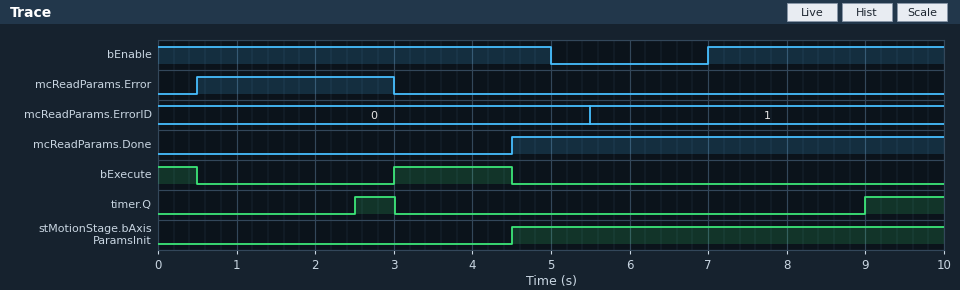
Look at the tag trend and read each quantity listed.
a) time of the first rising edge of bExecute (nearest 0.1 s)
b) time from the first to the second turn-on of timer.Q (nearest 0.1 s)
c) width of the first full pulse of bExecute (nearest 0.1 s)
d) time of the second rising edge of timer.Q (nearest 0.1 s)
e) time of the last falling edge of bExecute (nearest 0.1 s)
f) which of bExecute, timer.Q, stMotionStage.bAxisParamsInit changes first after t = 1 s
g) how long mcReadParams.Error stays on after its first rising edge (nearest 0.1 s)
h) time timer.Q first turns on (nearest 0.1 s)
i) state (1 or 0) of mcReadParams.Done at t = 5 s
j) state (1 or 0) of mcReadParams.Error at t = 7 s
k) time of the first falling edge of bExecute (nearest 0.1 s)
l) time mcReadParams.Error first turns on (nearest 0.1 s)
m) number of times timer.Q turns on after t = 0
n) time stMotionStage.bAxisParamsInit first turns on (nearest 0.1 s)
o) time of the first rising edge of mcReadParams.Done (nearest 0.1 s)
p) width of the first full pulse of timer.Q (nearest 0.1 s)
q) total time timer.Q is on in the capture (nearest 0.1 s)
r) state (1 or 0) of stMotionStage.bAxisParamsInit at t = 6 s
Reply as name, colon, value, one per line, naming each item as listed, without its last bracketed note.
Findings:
time of the first rising edge of bExecute: 3.0 s
time from the first to the second turn-on of timer.Q: 6.5 s
width of the first full pulse of bExecute: 1.5 s
time of the second rising edge of timer.Q: 9.0 s
time of the last falling edge of bExecute: 4.5 s
which of bExecute, timer.Q, stMotionStage.bAxisParamsInit changes first after t = 1 s: timer.Q
how long mcReadParams.Error stays on after its first rising edge: 2.5 s
time timer.Q first turns on: 2.5 s
state (1 or 0) of mcReadParams.Done at t = 5 s: 1
state (1 or 0) of mcReadParams.Error at t = 7 s: 0
time of the first falling edge of bExecute: 0.5 s
time mcReadParams.Error first turns on: 0.5 s
number of times timer.Q turns on after t = 0: 2
time stMotionStage.bAxisParamsInit first turns on: 4.5 s
time of the first rising edge of mcReadParams.Done: 4.5 s
width of the first full pulse of timer.Q: 0.5 s
total time timer.Q is on in the capture: 1.5 s
state (1 or 0) of stMotionStage.bAxisParamsInit at t = 6 s: 1
